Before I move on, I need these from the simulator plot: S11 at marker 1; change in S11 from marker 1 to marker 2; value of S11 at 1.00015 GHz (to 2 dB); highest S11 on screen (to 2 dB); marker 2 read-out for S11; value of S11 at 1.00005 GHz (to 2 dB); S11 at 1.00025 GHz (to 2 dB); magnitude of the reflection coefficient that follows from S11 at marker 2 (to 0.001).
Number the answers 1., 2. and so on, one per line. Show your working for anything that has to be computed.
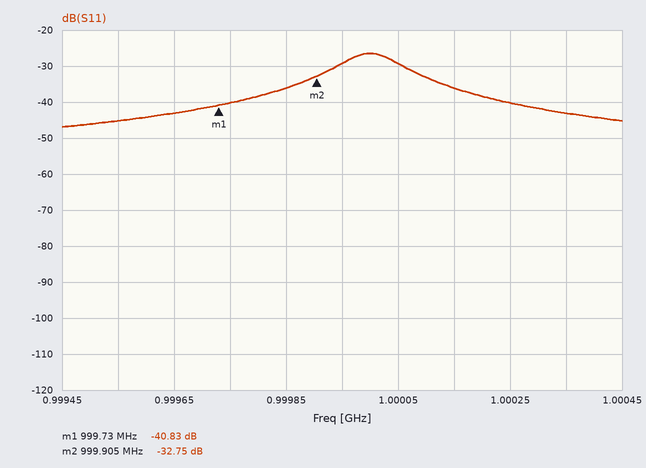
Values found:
1. -40.83 dB
2. -32.75 − (-40.83) = 8.08 dB
3. -36 dB
4. -26 dB
5. -32.75 dB
6. -30 dB
7. -40 dB
8. 10^(-32.75/20) ≈ 0.023
